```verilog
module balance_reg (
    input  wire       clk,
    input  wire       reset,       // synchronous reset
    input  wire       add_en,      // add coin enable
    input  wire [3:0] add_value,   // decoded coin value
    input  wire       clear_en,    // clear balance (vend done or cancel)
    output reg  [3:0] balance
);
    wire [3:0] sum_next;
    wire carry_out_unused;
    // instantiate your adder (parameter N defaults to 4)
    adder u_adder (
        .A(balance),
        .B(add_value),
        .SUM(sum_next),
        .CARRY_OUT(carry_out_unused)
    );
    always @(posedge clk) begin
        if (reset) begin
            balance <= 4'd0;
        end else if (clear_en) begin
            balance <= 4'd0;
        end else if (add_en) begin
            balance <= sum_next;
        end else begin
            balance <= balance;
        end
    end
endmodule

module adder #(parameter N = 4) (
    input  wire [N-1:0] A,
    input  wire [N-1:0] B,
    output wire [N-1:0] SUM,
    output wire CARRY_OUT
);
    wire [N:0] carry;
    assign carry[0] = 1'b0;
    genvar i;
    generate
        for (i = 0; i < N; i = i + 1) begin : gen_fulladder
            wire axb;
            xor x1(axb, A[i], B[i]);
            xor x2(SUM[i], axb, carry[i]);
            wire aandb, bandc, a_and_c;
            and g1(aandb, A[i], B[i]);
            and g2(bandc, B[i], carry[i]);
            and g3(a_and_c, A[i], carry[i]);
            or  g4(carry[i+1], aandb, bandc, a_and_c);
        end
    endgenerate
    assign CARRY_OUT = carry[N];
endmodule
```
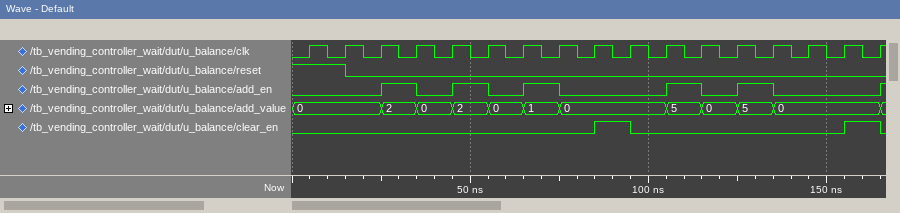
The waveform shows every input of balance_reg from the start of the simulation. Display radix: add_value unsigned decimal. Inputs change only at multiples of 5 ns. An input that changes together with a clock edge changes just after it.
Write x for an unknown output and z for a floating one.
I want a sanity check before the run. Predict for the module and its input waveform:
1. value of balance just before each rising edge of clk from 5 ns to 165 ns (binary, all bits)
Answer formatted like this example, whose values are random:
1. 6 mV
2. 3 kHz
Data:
1. x, 0000, 0000, 0000, 0010, 0010, 0100, 0100, 0101, 0101, 0000, 0000, 0101, 0101, 1010, 1010, 1010
